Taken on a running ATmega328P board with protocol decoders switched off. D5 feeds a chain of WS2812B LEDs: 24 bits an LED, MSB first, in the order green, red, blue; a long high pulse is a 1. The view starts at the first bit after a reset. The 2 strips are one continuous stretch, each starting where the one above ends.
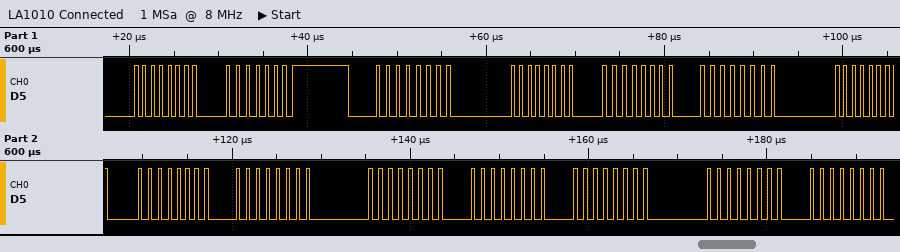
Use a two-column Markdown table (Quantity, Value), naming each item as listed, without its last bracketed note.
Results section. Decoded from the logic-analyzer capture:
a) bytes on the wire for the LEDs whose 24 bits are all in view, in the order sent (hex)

| Quantity | Value |
|---|---|
| bytes on the wire for the LEDs whose 24 bits are all in view, in the order sent | 00 01 00 00 00 00 00 00 00 00 00 00 |
